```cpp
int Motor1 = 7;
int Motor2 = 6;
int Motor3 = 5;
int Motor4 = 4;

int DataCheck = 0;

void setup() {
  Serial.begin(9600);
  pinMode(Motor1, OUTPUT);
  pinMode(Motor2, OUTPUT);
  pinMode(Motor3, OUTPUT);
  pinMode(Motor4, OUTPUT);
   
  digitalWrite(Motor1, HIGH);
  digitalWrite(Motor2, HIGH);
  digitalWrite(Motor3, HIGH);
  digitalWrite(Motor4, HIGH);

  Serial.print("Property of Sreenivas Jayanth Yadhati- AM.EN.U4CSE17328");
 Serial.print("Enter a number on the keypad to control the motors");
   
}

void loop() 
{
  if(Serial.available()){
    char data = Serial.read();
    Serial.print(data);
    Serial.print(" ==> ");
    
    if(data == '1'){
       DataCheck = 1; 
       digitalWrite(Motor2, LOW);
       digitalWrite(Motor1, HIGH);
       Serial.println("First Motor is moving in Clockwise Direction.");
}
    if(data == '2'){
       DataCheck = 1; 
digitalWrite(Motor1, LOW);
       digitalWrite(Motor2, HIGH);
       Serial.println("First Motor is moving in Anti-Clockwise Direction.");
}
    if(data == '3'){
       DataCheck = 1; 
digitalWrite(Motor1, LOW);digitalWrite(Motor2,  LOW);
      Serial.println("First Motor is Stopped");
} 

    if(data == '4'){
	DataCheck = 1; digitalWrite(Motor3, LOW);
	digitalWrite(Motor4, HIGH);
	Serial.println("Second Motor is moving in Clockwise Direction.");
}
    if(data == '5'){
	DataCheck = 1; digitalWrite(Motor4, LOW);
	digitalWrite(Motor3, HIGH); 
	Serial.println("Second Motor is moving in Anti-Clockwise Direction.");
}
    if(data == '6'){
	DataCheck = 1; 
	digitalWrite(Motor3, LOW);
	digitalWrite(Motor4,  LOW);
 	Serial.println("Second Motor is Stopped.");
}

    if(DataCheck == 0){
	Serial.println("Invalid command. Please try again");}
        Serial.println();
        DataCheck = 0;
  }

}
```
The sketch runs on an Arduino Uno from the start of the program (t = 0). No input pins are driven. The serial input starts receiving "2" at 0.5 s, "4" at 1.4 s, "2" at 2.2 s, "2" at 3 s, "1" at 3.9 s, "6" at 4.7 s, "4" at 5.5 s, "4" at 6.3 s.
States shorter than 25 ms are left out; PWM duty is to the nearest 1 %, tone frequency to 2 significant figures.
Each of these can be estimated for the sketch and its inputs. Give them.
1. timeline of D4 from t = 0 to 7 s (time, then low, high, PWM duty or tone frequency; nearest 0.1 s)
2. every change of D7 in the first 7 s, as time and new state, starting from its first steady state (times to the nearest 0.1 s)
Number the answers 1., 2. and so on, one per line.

1. 0 s high; 4.7 s low; 5.5 s high
2. 0 s high; 0.5 s low; 3.9 s high
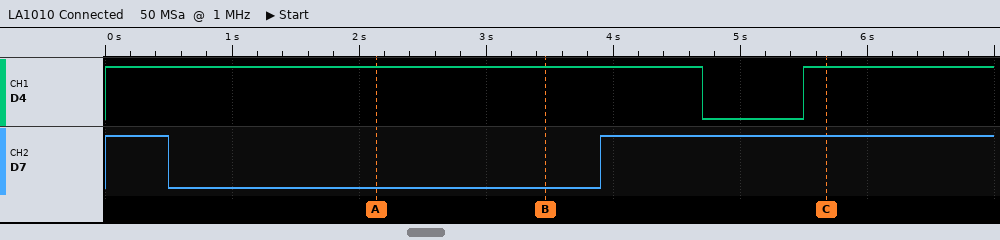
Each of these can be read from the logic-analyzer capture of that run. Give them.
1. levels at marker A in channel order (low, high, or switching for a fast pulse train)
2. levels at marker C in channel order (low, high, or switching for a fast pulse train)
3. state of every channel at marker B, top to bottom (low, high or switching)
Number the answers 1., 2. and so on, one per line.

1. D4 high, D7 low
2. D4 high, D7 high
3. D4 high, D7 low
